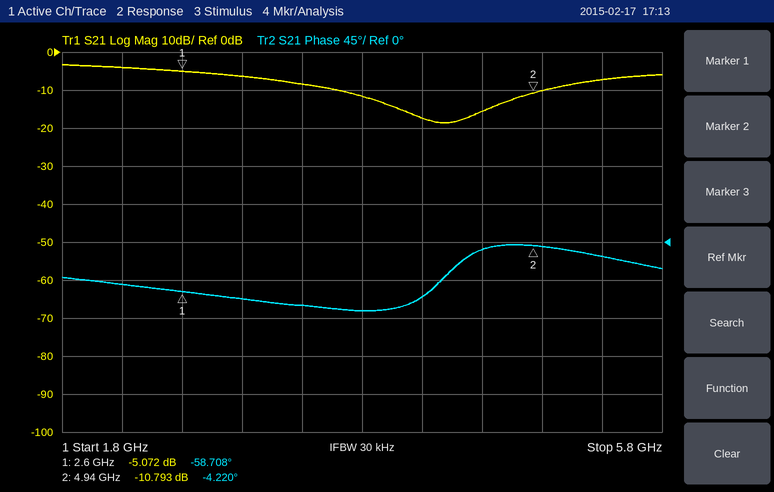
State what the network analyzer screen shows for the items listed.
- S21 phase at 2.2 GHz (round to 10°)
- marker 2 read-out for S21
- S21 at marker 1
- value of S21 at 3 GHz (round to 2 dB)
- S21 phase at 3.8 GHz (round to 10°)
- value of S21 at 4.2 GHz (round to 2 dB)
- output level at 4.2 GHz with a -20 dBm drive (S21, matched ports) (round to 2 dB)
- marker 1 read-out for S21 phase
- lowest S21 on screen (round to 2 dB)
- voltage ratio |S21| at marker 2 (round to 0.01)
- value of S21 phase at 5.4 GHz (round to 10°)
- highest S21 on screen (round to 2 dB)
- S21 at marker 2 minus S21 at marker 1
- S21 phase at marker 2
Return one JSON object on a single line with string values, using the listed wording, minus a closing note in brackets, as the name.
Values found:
{"S21 phase at 2.2 GHz": "-50°", "marker 2 read-out for S21": "-10.793 dB", "S21 at marker 1": "-5.072 dB", "value of S21 at 3 GHz": "-6 dB", "S21 phase at 3.8 GHz": "-80°", "value of S21 at 4.2 GHz": "-18 dB", "output level at 4.2 GHz with a -20 dBm drive (S21, matched ports)": "-38 dBm", "marker 1 read-out for S21 phase": "-58.708°", "lowest S21 on screen": "-18 dB", "voltage ratio |S21| at marker 2": "0.29", "value of S21 phase at 5.4 GHz": "-20°", "highest S21 on screen": "-4 dB", "S21 at marker 2 minus S21 at marker 1": "-5.721 dB", "S21 phase at marker 2": "-4.220°"}
